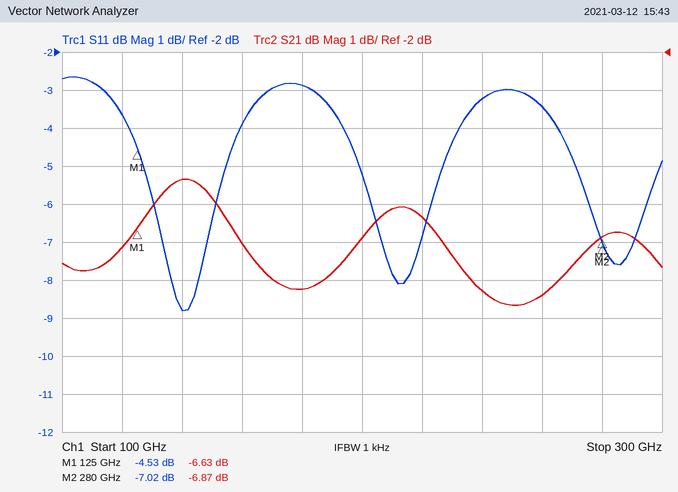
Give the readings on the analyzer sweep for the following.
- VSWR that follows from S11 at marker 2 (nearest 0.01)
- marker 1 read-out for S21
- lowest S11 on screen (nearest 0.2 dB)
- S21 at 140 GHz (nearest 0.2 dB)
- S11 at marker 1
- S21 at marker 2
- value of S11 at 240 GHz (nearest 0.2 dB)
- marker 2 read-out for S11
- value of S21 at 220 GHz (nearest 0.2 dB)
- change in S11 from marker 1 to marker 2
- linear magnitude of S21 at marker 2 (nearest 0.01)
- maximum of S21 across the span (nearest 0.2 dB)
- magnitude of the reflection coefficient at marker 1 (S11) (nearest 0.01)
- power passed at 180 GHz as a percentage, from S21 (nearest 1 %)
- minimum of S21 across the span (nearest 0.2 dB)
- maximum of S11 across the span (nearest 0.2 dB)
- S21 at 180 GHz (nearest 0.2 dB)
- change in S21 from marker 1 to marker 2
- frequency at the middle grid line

2.61
-6.63 dB
-8.8 dB
-5.4 dB
-4.53 dB
-6.87 dB
-3.2 dB
-7.02 dB
-6.4 dB
-2.49 dB
0.45
-5.4 dB
0.59
15 %
-8.6 dB
-2.6 dB
-8.2 dB
-0.24 dB
200 GHz
